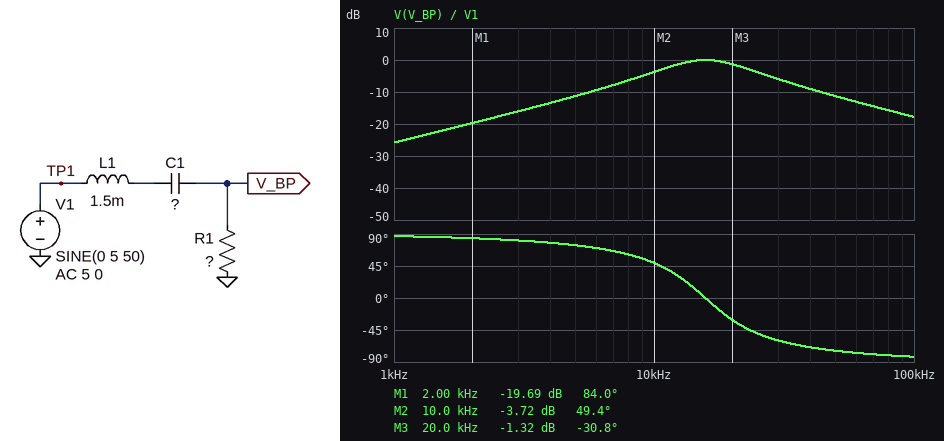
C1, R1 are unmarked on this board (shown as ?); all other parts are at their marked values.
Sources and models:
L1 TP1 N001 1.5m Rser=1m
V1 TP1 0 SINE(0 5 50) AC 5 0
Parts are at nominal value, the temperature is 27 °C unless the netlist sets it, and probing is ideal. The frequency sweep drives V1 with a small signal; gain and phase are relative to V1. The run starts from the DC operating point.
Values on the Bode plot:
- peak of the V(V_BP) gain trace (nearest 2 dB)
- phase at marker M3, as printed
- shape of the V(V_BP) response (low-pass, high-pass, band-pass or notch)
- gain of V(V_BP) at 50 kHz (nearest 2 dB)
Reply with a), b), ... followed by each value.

a) 0 dB
b) -30.8 deg
c) band-pass
d) -12 dB
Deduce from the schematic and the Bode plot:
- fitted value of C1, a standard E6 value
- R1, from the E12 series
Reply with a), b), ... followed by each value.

a) 68 nF
b) 120 Ω
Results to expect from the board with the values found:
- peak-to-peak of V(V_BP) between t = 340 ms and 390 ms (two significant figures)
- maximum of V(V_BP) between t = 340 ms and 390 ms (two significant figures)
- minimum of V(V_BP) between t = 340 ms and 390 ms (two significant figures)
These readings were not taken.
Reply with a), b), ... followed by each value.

a) 26 mV
b) 13 mV
c) -13 mV
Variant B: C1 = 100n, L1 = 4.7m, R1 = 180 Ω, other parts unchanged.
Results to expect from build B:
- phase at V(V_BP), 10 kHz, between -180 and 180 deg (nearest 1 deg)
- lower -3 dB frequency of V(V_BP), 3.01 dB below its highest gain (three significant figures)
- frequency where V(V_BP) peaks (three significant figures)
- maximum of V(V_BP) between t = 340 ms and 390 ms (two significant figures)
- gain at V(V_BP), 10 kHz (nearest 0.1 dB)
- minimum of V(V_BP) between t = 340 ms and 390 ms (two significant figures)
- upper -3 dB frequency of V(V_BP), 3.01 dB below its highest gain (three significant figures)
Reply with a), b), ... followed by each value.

a) -37 deg
b) 4.90 kHz
c) 7.34 kHz
d) 28 mV
e) -2.0 dB
f) -28 mV
g) 11.0 kHz
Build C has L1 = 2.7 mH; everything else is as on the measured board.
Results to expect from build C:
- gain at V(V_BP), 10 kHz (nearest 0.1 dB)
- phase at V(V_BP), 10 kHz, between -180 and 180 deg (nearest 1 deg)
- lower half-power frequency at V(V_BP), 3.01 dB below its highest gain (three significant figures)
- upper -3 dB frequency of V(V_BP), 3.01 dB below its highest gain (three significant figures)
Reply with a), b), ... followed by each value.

a) -1.1 dB
b) 28 deg
c) 8.73 kHz
d) 15.8 kHz
